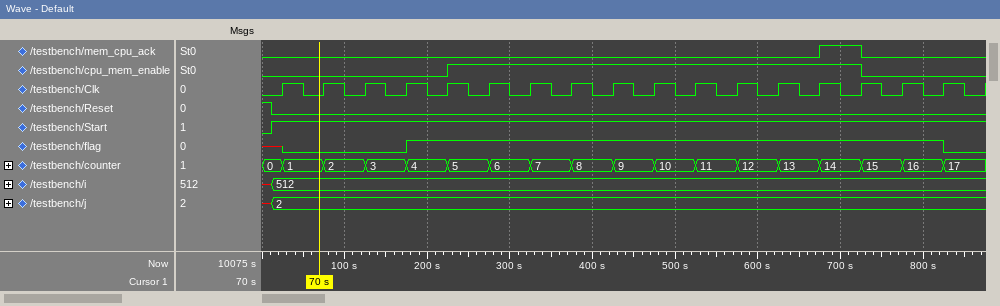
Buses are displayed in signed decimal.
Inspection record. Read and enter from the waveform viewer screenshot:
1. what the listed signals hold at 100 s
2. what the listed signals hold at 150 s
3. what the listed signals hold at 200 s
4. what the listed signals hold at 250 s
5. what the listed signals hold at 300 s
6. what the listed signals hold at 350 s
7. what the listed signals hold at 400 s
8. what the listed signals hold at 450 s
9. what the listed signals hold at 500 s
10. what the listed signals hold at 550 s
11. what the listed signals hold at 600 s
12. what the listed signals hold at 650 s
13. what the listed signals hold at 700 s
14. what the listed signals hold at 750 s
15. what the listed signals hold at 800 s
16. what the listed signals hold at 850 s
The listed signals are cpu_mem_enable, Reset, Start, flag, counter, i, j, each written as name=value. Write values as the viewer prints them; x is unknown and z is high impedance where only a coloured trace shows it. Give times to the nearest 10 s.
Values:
cpu_mem_enable=0, Reset=0, Start=1, flag=0, counter=2, i=512, j=2
cpu_mem_enable=0, Reset=0, Start=1, flag=0, counter=3, i=512, j=2
cpu_mem_enable=0, Reset=0, Start=1, flag=1, counter=4, i=512, j=2
cpu_mem_enable=1, Reset=0, Start=1, flag=1, counter=5, i=512, j=2
cpu_mem_enable=1, Reset=0, Start=1, flag=1, counter=6, i=512, j=2
cpu_mem_enable=1, Reset=0, Start=1, flag=1, counter=7, i=512, j=2
cpu_mem_enable=1, Reset=0, Start=1, flag=1, counter=8, i=512, j=2
cpu_mem_enable=1, Reset=0, Start=1, flag=1, counter=9, i=512, j=2
cpu_mem_enable=1, Reset=0, Start=1, flag=1, counter=10, i=512, j=2
cpu_mem_enable=1, Reset=0, Start=1, flag=1, counter=11, i=512, j=2
cpu_mem_enable=1, Reset=0, Start=1, flag=1, counter=12, i=512, j=2
cpu_mem_enable=1, Reset=0, Start=1, flag=1, counter=13, i=512, j=2
cpu_mem_enable=1, Reset=0, Start=1, flag=1, counter=14, i=512, j=2
cpu_mem_enable=0, Reset=0, Start=1, flag=1, counter=15, i=512, j=2
cpu_mem_enable=0, Reset=0, Start=1, flag=1, counter=16, i=512, j=2
cpu_mem_enable=0, Reset=0, Start=1, flag=0, counter=17, i=512, j=2
